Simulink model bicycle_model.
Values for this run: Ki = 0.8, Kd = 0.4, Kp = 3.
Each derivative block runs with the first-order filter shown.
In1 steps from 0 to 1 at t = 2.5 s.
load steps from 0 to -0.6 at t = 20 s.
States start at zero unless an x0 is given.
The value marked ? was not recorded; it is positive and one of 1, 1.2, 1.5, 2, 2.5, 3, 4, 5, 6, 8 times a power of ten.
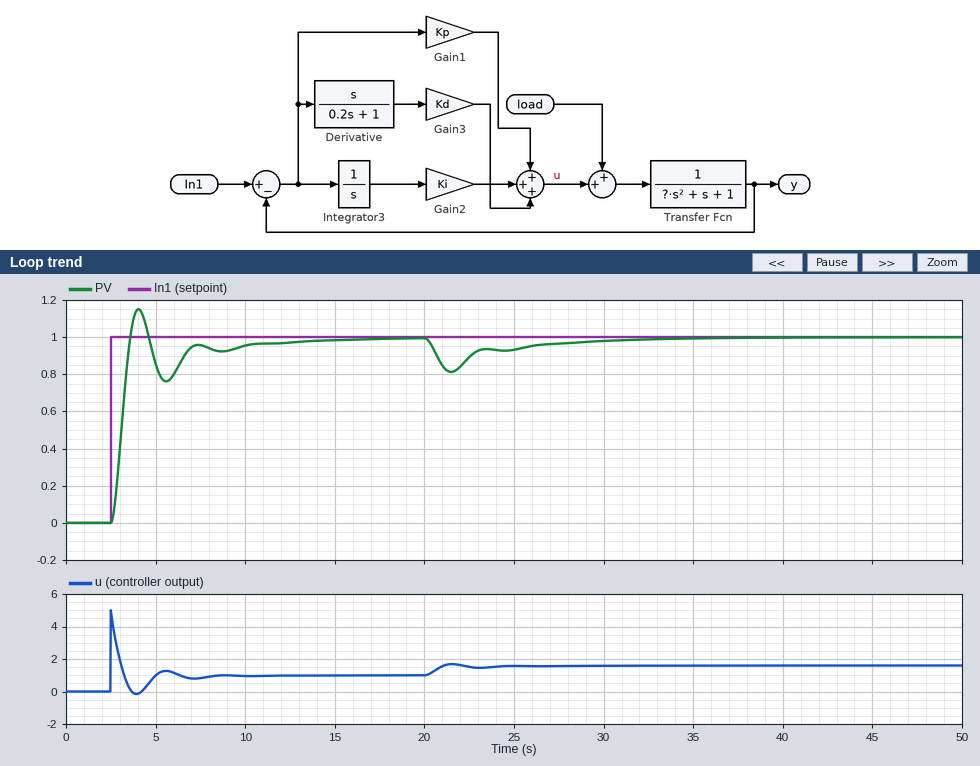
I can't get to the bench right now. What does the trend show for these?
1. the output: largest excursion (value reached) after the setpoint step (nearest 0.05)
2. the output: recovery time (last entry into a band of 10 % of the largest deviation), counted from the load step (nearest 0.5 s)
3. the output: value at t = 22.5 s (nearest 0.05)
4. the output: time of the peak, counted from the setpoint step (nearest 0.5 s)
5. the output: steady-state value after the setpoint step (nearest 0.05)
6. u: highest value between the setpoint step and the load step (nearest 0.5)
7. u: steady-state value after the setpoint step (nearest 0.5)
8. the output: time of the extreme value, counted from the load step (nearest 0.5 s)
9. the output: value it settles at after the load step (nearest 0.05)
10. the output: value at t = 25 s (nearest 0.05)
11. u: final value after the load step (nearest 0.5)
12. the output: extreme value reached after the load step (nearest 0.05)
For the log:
1.15
10.5 s
0.90
1.5 s
1.00
5.0
1.0
1.5 s
1.00
0.95
1.5
0.80
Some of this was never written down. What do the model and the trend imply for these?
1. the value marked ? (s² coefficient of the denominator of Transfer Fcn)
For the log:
1
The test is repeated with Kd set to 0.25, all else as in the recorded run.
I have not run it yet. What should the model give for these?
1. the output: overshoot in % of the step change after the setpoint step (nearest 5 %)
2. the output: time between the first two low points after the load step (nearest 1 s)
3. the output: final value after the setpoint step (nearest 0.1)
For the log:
20 %
3 s
1.0
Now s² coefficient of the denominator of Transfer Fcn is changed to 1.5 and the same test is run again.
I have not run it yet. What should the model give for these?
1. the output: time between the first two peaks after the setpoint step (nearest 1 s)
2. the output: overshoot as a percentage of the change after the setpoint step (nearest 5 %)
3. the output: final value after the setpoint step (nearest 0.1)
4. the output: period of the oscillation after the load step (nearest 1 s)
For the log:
4 s
25 %
1.0
4 s
